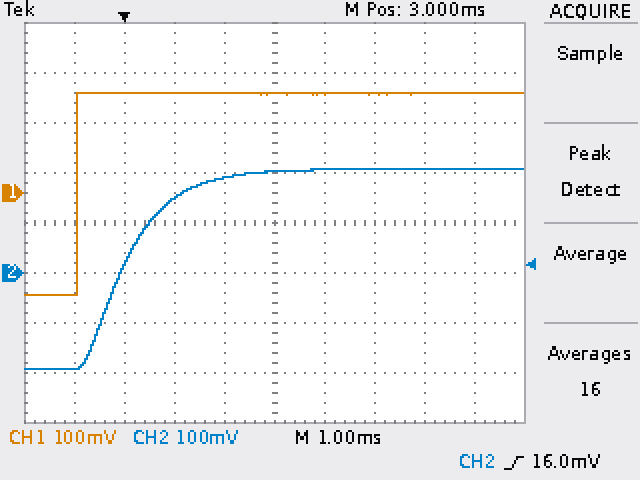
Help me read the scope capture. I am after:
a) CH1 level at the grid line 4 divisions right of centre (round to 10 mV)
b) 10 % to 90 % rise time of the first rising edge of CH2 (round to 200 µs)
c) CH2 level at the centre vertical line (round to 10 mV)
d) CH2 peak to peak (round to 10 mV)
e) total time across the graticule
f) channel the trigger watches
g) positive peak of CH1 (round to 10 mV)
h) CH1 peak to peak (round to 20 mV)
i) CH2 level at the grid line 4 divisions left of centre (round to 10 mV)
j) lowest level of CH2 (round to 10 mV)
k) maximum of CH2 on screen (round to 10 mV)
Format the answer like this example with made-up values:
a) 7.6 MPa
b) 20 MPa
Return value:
a) 200 mV
b) 2.0 ms
c) 200 mV
d) 400 mV
e) 10 ms
f) CH2
g) 200 mV
h) 400 mV
i) -190 mV
j) -190 mV
k) 210 mV
